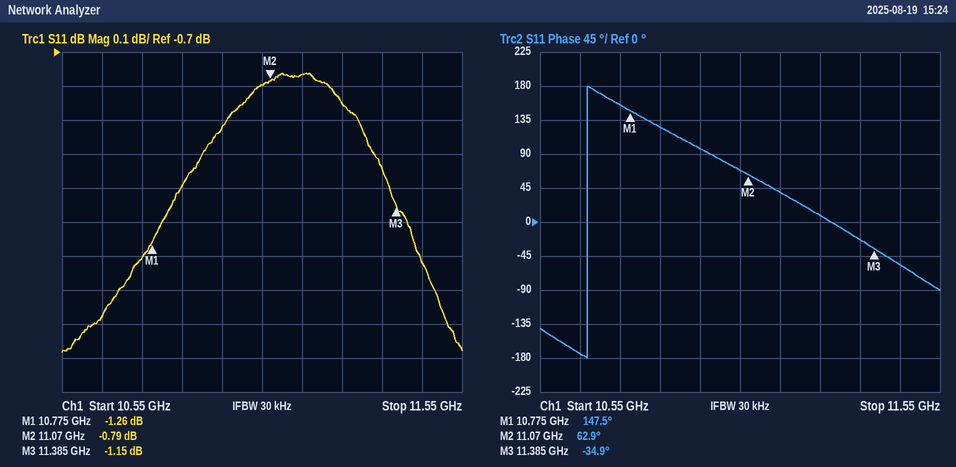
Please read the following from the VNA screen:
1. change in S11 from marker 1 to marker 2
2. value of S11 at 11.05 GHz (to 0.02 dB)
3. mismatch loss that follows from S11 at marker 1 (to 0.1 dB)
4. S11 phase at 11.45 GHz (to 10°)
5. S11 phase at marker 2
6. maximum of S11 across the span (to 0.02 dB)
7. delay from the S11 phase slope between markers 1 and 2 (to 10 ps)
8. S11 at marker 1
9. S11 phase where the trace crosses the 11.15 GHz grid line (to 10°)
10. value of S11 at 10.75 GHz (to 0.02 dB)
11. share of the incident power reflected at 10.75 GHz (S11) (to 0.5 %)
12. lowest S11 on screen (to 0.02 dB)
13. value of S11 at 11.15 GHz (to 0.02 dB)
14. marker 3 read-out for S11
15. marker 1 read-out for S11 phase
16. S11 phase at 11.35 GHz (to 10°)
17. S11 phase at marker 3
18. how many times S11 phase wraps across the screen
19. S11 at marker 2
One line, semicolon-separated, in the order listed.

0.47 dB; -0.80 dB; 6.0 dB; -60°; 62.9°; -0.76 dB; 800 ps; -1.26 dB; 40°; -1.30 dB; 74.0 %; -1.58 dB; -0.76 dB; -1.15 dB; 147.5°; -20°; -34.9°; 1; -0.79 dB
